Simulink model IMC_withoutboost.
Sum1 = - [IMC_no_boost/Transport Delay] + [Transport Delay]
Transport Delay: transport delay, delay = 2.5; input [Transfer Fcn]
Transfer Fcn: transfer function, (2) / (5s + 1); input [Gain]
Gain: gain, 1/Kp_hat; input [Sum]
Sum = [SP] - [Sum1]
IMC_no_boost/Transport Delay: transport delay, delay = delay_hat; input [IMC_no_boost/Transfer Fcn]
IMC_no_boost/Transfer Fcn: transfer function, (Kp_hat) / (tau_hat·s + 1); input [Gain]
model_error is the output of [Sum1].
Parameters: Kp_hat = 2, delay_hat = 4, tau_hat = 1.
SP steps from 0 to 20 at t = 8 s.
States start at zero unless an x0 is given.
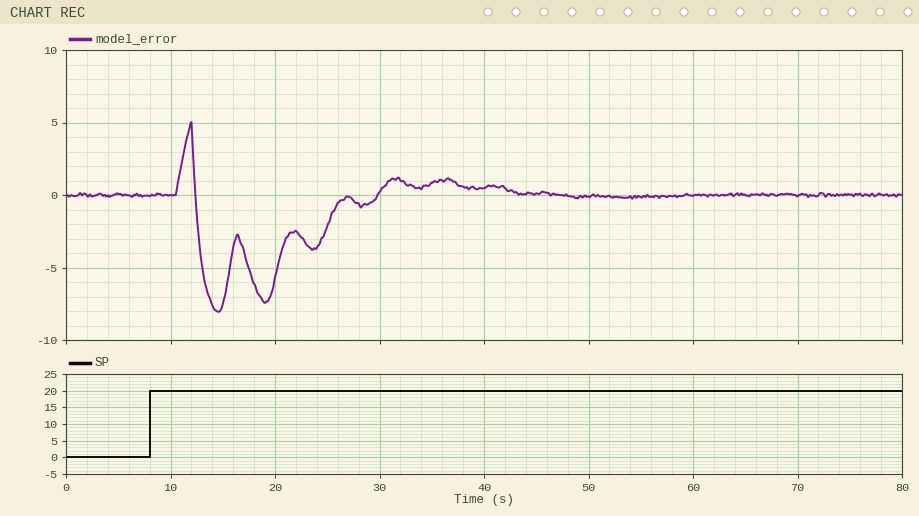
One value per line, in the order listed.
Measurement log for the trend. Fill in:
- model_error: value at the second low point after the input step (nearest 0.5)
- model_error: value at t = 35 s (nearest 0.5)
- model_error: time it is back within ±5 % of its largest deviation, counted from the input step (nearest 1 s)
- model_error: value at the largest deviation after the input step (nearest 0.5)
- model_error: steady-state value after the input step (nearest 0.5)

-7.5
1.0
34 s
-8.0
0.0
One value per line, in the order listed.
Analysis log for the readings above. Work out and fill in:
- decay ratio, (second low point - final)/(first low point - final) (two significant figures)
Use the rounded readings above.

0.94
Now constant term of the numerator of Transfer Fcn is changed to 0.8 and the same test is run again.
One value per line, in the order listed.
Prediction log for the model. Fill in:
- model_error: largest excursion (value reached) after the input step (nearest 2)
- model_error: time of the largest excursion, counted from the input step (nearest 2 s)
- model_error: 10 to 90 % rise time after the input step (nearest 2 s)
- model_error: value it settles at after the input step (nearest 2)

-32
30 s
10 s
-30
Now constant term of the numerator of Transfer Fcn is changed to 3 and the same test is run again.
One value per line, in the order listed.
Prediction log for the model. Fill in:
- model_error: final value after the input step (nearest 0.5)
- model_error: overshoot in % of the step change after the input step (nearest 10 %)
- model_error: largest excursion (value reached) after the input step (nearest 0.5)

6.5
40 %
9.0
